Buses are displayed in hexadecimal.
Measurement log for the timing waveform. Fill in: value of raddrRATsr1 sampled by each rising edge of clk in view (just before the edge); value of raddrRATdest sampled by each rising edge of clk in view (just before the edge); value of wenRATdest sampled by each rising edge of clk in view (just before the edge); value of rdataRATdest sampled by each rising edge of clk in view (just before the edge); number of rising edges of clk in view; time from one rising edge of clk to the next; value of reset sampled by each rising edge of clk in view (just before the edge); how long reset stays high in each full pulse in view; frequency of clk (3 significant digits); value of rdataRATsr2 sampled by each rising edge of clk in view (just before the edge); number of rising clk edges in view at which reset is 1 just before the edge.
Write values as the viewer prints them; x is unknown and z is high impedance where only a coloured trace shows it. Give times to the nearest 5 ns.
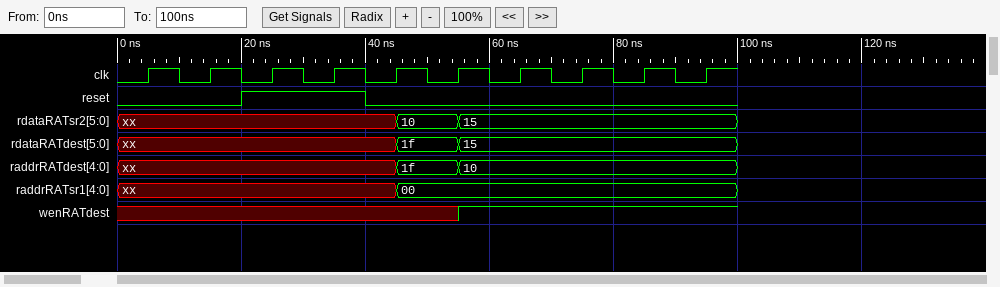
xx, xx, xx, xx, xx, 00, 00, 00, 00, 00
xx, xx, xx, xx, xx, 1f, 10, 10, 10, 10
x x x x x x 1 1 1 1
xx, xx, xx, xx, xx, 1f, 15, 15, 15, 15
10
10 ns
0 0 1 1 0 0 0 0 0 0
20 ns
100 MHz
xx, xx, xx, xx, xx, 10, 15, 15, 15, 15
2
